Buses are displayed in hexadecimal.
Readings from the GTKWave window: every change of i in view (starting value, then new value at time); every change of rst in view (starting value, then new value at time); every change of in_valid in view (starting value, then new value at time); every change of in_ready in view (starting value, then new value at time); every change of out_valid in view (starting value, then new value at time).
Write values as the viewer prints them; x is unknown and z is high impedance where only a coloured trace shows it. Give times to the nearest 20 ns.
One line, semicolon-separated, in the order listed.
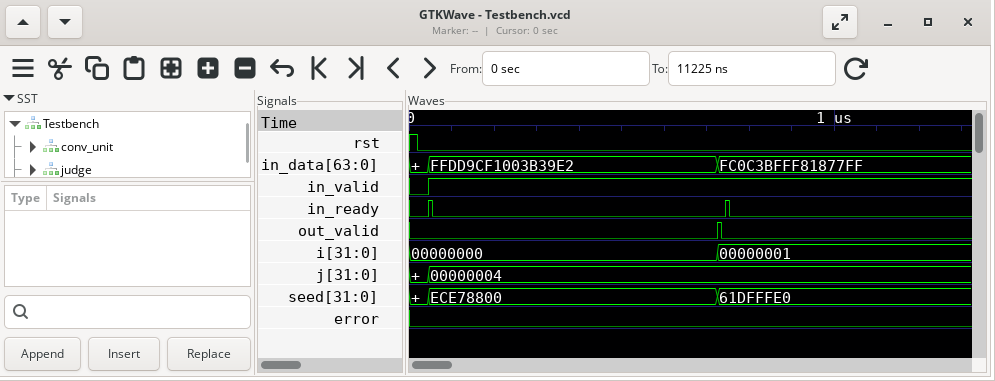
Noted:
00000000, 00000001 at 720 ns; 1, 0 at 20 ns; 0, 1 at 40 ns; 0, 1 at 40 ns, 0 at 60 ns, 1 at 740 ns, 0 at 760 ns; 0, 1 at 720 ns, 0 at 740 ns
